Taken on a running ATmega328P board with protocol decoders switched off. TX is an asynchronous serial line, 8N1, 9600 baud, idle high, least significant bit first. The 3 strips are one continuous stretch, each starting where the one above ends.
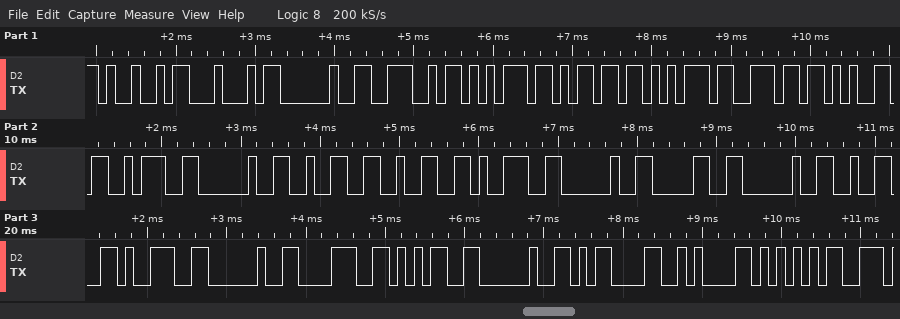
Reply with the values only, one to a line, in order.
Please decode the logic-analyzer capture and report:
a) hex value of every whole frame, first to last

49 44 20 4E 75 6D 75 6E 65 3A 20 32 32 39 20 30 20 32 39 20 38 35 20 0D 0A 55
